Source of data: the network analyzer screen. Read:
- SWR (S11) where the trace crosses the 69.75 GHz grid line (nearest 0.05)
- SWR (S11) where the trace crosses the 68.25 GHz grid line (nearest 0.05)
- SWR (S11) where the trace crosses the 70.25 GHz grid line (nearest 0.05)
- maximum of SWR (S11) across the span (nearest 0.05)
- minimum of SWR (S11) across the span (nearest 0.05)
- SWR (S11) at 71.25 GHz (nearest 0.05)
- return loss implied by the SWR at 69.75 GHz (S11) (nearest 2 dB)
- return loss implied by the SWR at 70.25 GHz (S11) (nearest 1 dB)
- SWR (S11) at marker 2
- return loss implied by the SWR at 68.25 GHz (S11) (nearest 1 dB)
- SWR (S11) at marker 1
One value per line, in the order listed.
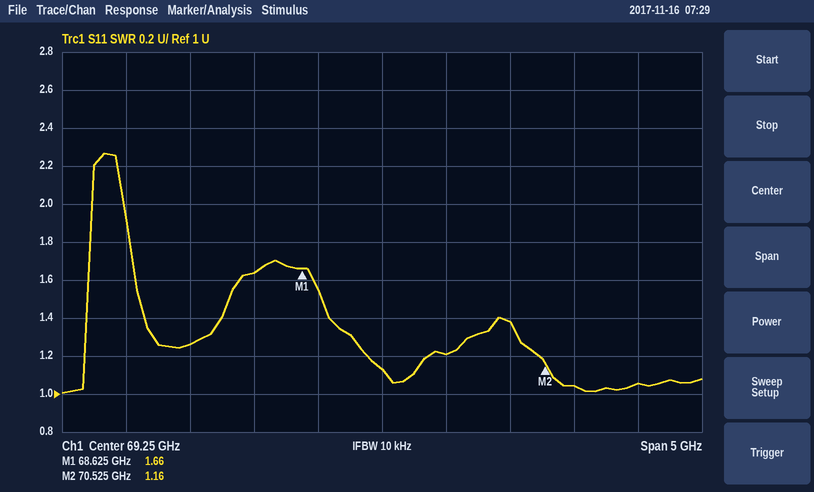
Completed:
1.20
1.65
1.40
2.25
1.00
1.05
20 dB
16 dB
1.16
12 dB
1.66
